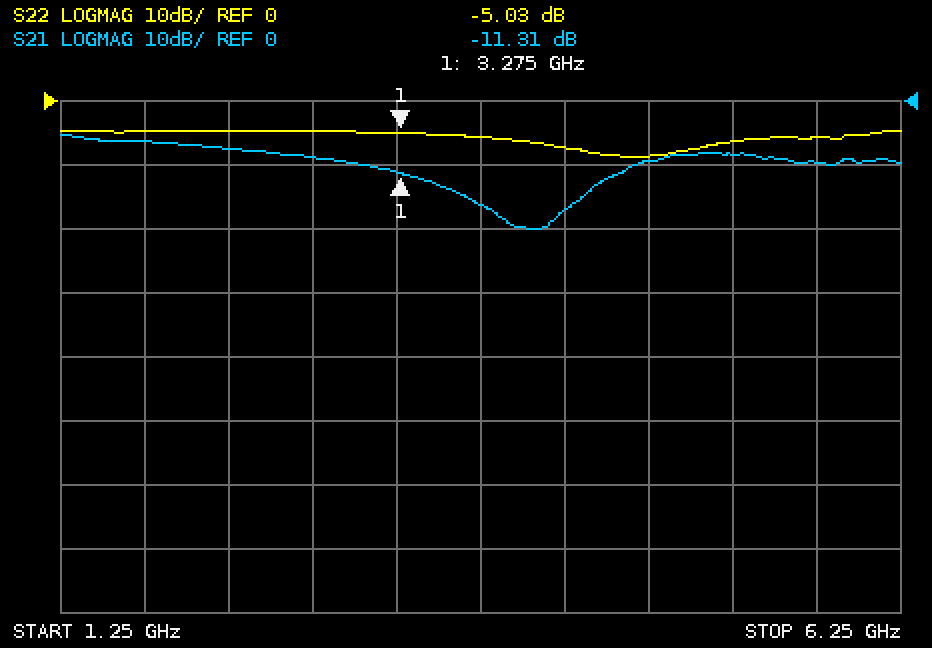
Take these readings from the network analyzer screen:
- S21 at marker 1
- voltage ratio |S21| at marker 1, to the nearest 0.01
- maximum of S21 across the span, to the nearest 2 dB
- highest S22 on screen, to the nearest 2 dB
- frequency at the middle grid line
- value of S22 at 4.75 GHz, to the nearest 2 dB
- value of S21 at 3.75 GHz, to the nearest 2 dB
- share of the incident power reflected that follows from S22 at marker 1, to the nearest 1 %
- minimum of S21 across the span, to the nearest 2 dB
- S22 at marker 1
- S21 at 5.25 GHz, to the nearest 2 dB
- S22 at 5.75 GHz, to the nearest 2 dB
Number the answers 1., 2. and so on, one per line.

1. -11.31 dB
2. 0.27
3. -6 dB
4. -4 dB
5. 3.75 GHz
6. -8 dB
7. -16 dB
8. 31 %
9. -20 dB
10. -5.03 dB
11. -8 dB
12. -6 dB
